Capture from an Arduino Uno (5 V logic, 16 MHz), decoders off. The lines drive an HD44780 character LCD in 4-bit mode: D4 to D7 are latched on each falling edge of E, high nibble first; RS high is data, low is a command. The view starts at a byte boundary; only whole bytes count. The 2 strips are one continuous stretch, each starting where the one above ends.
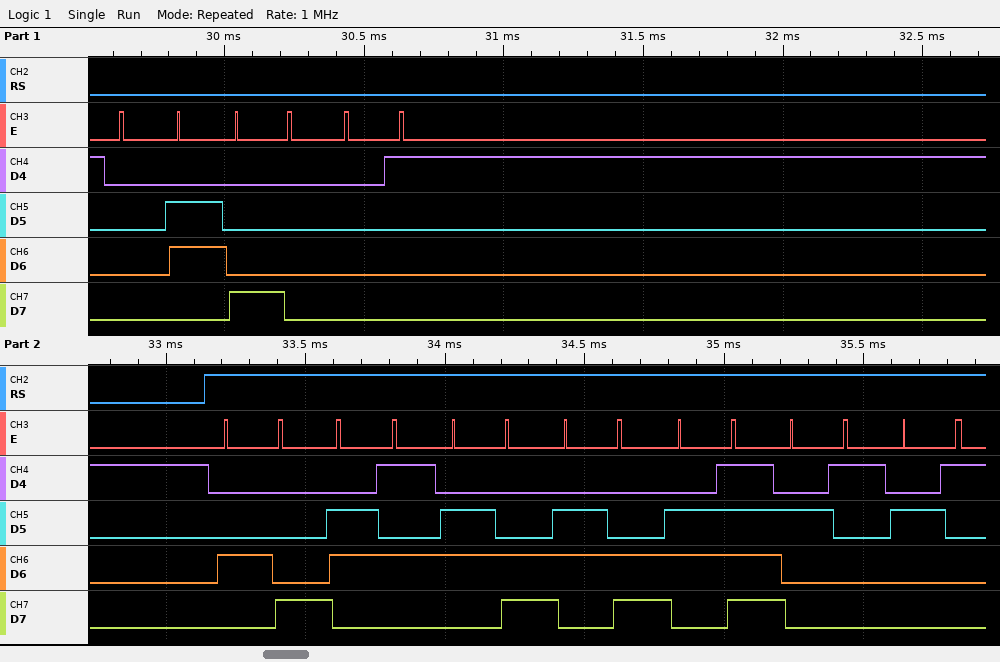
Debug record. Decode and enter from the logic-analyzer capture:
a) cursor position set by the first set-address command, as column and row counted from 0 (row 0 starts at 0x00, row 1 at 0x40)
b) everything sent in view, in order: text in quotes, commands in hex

column 0, row 0
0x06 0x80 0x01 "Hello!!"
